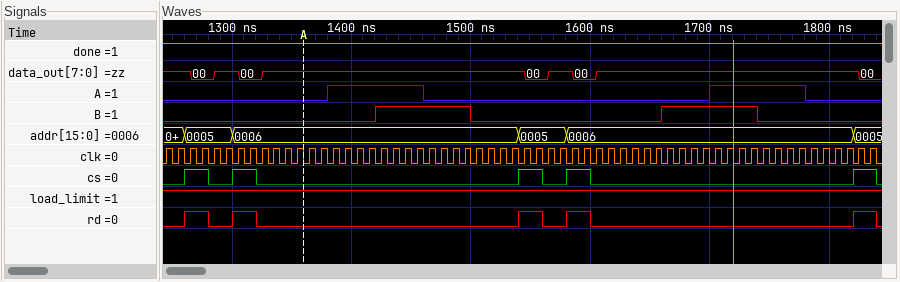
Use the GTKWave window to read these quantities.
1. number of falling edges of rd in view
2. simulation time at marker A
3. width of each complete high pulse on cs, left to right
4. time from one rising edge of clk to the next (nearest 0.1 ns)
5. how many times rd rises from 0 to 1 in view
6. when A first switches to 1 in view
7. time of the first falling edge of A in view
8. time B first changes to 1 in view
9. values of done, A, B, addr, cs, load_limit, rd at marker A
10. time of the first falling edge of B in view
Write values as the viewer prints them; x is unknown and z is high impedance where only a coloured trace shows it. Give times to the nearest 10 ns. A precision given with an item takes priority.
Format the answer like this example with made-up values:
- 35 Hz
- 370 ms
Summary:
- 5
- 1360 ns
- 20 ns, 20 ns, 20 ns, 20 ns, 20 ns
- 10 ns
- 5
- 1380 ns
- 1460 ns
- 1420 ns
- done=1, A=0, B=0, addr=0006, cs=0, load_limit=1, rd=0
- 1500 ns
